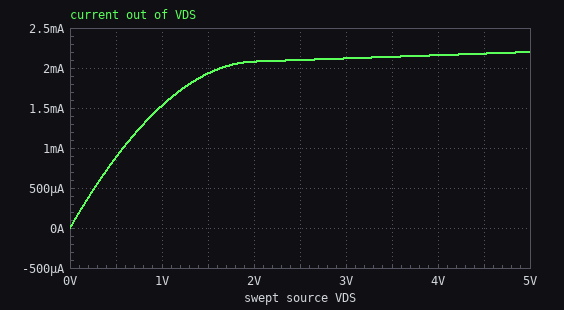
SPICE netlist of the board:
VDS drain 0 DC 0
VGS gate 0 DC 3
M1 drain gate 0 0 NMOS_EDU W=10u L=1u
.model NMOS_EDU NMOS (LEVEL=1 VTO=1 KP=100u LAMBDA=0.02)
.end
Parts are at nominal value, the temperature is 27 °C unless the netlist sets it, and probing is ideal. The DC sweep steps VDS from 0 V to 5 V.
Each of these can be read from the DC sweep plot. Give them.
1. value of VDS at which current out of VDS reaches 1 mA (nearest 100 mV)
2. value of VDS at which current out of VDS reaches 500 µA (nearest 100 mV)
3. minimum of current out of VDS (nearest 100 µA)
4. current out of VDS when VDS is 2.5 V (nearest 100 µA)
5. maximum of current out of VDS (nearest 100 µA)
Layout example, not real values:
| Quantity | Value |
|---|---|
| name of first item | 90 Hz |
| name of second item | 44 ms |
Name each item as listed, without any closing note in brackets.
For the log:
| Quantity | Value |
|---|---|
| value of VDS at which current out of VDS reaches 1 mA | 600 mV |
| value of VDS at which current out of VDS reaches 500 µA | 300 mV |
| minimum of current out of VDS | 0 A |
| current out of VDS when VDS is 2.5 V | 2.1 mA |
| maximum of current out of VDS | 2.2 mA |
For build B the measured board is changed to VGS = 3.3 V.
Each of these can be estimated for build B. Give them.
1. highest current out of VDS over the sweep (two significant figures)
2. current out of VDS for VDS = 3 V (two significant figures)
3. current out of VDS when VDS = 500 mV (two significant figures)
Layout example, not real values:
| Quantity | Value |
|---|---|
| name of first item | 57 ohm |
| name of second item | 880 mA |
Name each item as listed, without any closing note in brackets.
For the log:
| Quantity | Value |
|---|---|
| highest current out of VDS over the sweep | 2.9 mA |
| current out of VDS for VDS = 3 V | 2.8 mA |
| current out of VDS when VDS = 500 mV | 1.0 mA |
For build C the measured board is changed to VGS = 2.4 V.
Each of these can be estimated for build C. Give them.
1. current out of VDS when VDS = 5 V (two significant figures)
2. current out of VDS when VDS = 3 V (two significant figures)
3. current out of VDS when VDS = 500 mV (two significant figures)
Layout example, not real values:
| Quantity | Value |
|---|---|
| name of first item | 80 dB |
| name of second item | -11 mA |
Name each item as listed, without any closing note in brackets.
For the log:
| Quantity | Value |
|---|---|
| current out of VDS when VDS = 5 V | 1.1 mA |
| current out of VDS when VDS = 3 V | 1.0 mA |
| current out of VDS when VDS = 500 mV | 580 µA |
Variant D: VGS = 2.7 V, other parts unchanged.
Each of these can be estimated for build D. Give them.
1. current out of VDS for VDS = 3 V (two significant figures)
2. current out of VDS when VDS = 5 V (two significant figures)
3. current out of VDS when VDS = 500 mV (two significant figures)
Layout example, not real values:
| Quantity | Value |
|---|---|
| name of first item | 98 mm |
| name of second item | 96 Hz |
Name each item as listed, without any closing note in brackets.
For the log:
| Quantity | Value |
|---|---|
| current out of VDS for VDS = 3 V | 1.5 mA |
| current out of VDS when VDS = 5 V | 1.6 mA |
| current out of VDS when VDS = 500 mV | 730 µA |
